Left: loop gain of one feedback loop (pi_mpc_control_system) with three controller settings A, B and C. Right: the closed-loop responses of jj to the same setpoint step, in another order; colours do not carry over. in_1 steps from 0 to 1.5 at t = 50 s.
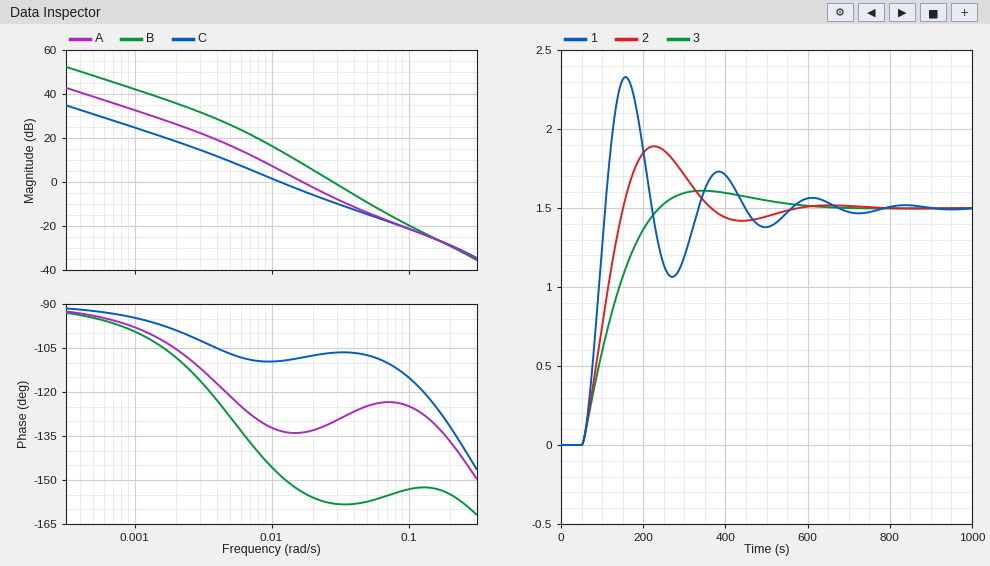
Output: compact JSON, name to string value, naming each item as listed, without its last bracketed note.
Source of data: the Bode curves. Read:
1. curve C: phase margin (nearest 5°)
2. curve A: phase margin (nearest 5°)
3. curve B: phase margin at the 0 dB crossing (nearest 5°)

{"curve C: phase margin": "70°", "curve A: phase margin": "45°", "curve B: phase margin at the 0 dB crossing": "20°"}
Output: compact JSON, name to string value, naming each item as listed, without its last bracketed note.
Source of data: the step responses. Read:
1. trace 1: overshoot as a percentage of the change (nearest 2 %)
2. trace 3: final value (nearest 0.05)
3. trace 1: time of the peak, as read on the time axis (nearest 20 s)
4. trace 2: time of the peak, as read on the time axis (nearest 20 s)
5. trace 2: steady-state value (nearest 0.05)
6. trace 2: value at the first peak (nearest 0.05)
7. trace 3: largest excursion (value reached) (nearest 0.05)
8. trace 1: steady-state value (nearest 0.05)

{"trace 1: overshoot as a percentage of the change": "56 %", "trace 3: final value": "1.50", "trace 1: time of the peak, as read on the time axis": "160 s", "trace 2: time of the peak, as read on the time axis": "220 s", "trace 2: steady-state value": "1.50", "trace 2: value at the first peak": "1.90", "trace 3: largest excursion (value reached)": "1.60", "trace 1: steady-state value": "1.50"}
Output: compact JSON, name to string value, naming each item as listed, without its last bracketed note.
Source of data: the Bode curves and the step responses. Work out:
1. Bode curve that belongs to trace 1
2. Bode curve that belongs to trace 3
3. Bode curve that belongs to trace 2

{"Bode curve that belongs to trace 1": "B", "Bode curve that belongs to trace 3": "C", "Bode curve that belongs to trace 2": "A"}
